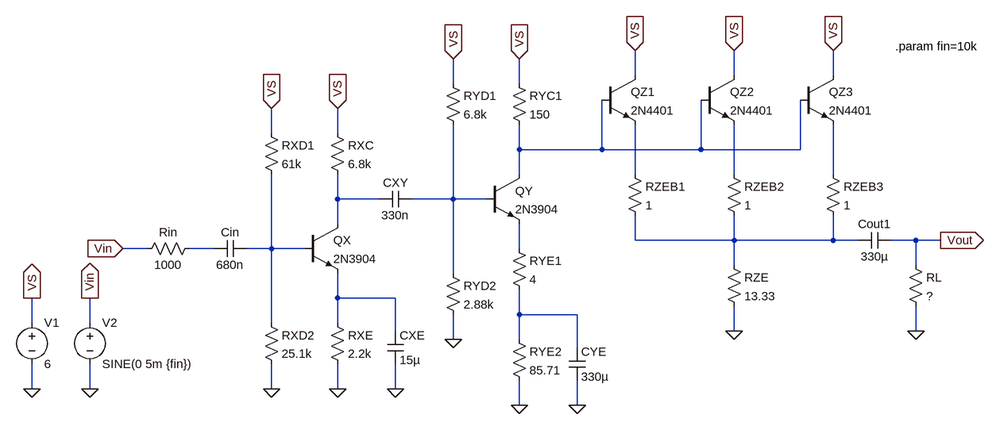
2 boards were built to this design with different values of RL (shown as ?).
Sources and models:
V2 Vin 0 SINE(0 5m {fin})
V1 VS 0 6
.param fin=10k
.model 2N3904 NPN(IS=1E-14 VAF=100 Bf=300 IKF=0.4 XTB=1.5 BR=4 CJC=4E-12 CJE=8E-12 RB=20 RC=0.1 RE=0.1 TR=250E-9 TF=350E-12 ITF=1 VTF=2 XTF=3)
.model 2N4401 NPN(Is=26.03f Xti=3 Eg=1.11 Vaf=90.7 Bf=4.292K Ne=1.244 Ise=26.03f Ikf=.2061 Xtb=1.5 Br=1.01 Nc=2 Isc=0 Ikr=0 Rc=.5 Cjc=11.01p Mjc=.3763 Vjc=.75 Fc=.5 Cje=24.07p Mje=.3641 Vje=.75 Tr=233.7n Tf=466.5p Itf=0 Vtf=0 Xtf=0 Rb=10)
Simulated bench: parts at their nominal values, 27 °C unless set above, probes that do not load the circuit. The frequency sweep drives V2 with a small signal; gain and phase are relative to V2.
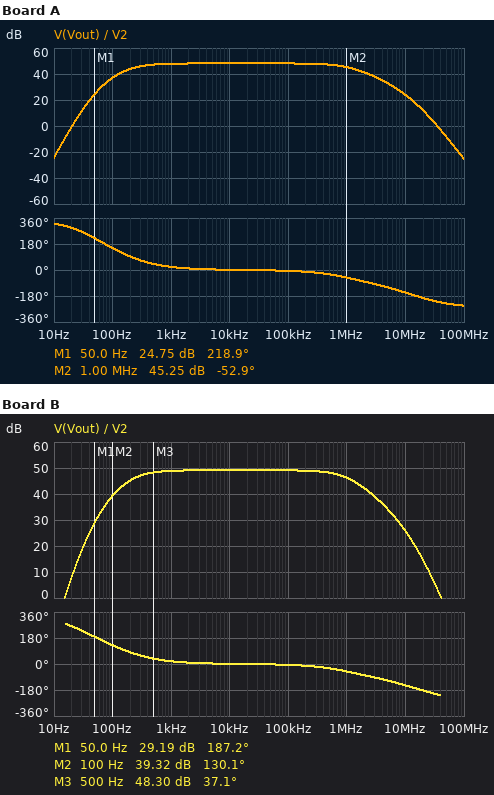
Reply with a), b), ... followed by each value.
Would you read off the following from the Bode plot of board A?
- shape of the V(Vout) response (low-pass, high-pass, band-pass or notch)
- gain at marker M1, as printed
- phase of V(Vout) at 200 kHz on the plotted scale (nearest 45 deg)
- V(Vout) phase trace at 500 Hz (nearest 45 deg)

a) band-pass
b) 24.75 dB
c) 0 deg
d) 45 deg
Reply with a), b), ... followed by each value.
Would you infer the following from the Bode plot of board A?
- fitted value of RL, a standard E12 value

a) 6.8 Ω
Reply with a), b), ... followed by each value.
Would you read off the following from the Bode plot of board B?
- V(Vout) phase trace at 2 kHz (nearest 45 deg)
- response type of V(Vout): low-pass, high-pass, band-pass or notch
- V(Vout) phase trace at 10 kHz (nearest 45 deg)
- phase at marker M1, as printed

a) 0 deg
b) band-pass
c) 0 deg
d) 187.2 deg
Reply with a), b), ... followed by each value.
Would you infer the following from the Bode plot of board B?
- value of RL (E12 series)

a) 27 Ω
